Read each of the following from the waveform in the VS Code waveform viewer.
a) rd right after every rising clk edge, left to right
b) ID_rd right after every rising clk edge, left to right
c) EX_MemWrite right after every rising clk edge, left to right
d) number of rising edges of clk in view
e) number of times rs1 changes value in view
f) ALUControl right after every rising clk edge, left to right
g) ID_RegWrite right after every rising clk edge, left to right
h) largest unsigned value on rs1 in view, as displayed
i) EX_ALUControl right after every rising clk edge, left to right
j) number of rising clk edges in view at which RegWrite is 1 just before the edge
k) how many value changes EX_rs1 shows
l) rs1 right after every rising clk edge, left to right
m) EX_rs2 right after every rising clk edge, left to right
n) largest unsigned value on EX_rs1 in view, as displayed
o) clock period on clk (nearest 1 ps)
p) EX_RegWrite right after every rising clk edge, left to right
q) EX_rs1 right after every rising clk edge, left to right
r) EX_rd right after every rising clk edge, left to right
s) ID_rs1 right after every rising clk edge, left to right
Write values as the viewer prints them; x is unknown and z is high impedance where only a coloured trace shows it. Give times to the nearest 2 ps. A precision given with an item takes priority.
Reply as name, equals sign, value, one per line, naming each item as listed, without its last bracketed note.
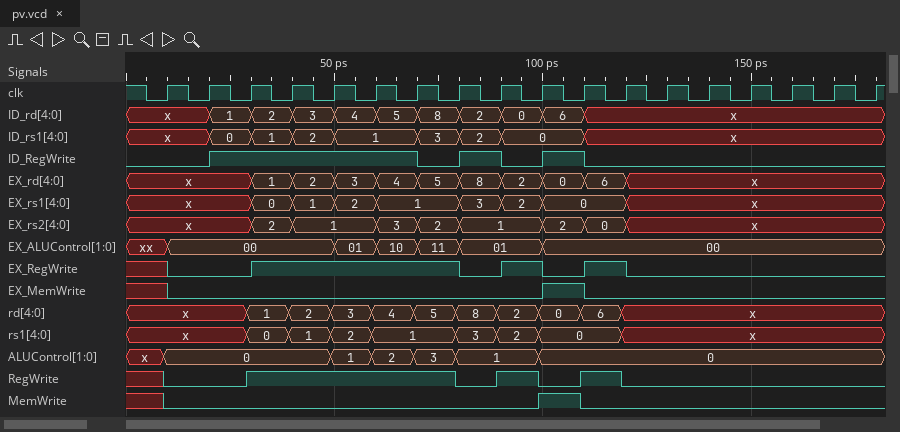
rd right after every rising clk edge, left to right = x, x, 1, 2, 3, 4, 5, 8, 2, 0, 6, x, x, x, x, x, x, x
ID_rd right after every rising clk edge, left to right = x, 1, 2, 3, 4, 5, 8, 2, 0, 6, x, x, x, x, x, x, x, x
EX_MemWrite right after every rising clk edge, left to right = 0 0 0 0 0 0 0 0 0 1 0 0 0 0 0 0 0 0
number of rising edges of clk in view = 18
number of times rs1 changes value in view = 8
ALUControl right after every rising clk edge, left to right = 0, 0, 0, 0, 1, 2, 3, 1, 1, 0, 0, 0, 0, 0, 0, 0, 0, 0
ID_RegWrite right after every rising clk edge, left to right = 0 1 1 1 1 1 0 1 0 1 0 0 0 0 0 0 0 0
largest unsigned value on rs1 in view, as displayed = 3
EX_ALUControl right after every rising clk edge, left to right = 00, 00, 00, 00, 01, 10, 11, 01, 01, 00, 00, 00, 00, 00, 00, 00, 00, 00
number of rising clk edges in view at which RegWrite is 1 just before the edge = 7
how many value changes EX_rs1 shows = 8
rs1 right after every rising clk edge, left to right = x, x, 0, 1, 2, 1, 1, 3, 2, 0, 0, x, x, x, x, x, x, x
EX_rs2 right after every rising clk edge, left to right = x, x, 2, 1, 1, 3, 2, 1, 1, 2, 0, x, x, x, x, x, x, x
largest unsigned value on EX_rs1 in view, as displayed = 3
clock period on clk = 10 ps
EX_RegWrite right after every rising clk edge, left to right = 0 0 1 1 1 1 1 0 1 0 1 0 0 0 0 0 0 0
EX_rs1 right after every rising clk edge, left to right = x, x, 0, 1, 2, 1, 1, 3, 2, 0, 0, x, x, x, x, x, x, x
EX_rd right after every rising clk edge, left to right = x, x, 1, 2, 3, 4, 5, 8, 2, 0, 6, x, x, x, x, x, x, x
ID_rs1 right after every rising clk edge, left to right = x, 0, 1, 2, 1, 1, 3, 2, 0, 0, x, x, x, x, x, x, x, x
